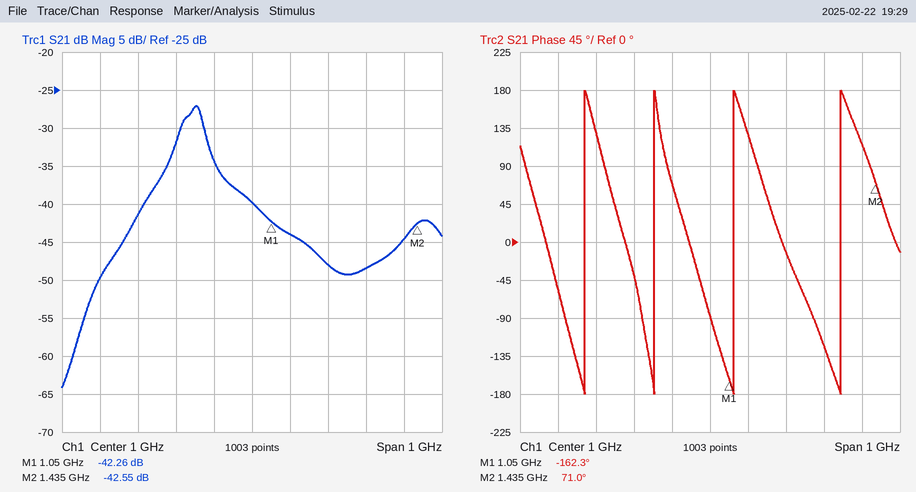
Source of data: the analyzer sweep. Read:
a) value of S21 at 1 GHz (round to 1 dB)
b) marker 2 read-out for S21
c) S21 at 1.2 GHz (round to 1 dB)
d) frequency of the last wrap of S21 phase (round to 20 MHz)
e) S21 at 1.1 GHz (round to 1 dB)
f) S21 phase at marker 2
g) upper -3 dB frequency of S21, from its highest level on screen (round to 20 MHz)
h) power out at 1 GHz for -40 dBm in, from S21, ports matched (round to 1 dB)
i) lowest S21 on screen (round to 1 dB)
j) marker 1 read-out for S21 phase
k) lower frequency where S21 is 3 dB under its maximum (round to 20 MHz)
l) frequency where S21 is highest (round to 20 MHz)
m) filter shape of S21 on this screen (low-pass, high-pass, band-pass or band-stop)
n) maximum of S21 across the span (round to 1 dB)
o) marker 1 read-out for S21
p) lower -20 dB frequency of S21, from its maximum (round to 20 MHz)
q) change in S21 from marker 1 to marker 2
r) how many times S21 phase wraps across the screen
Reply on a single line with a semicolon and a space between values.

-40 dB; -42.55 dB; -48 dB; 1.34 GHz; -44 dB; 71.0°; 880 MHz; -80 dBm; -64 dB; -162.3°; 820 MHz; 860 MHz; band-pass; -27 dB; -42.26 dB; 640 MHz; -0.29 dB; 4
